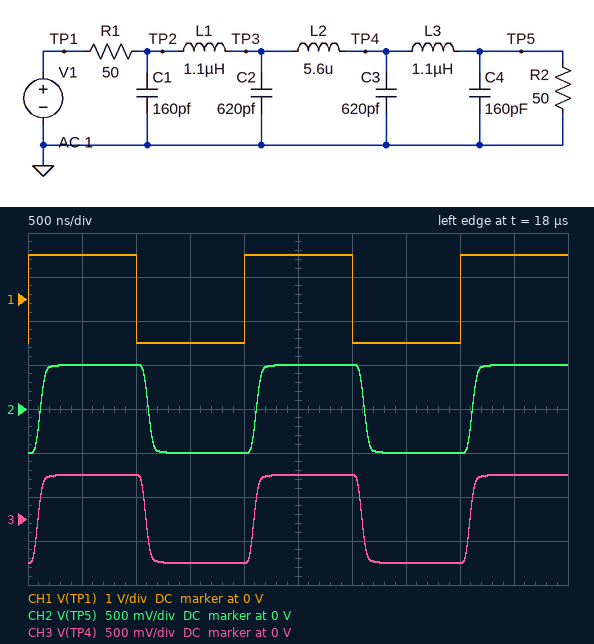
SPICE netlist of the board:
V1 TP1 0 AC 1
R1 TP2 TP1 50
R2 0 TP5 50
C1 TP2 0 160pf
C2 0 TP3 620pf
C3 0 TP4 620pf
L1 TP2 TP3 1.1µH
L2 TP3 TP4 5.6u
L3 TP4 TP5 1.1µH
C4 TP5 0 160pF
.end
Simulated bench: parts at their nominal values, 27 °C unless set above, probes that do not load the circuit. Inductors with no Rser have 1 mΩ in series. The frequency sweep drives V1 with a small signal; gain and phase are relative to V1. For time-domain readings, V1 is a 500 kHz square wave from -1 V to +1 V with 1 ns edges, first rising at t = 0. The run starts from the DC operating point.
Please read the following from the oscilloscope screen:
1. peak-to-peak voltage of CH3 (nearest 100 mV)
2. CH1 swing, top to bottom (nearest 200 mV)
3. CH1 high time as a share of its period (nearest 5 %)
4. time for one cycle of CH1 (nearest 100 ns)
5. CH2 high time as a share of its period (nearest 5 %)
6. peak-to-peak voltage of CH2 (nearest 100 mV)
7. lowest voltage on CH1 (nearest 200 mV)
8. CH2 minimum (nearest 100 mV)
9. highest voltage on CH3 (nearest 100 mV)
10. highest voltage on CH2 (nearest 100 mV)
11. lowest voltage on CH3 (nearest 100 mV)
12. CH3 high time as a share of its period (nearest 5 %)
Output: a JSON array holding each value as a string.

["1.0 V", "2.0 V", "50 %", "2.0 µs", "50 %", "1.0 V", "-1.0 V", "-500 mV", "500 mV", "500 mV", "-500 mV", "50 %"]
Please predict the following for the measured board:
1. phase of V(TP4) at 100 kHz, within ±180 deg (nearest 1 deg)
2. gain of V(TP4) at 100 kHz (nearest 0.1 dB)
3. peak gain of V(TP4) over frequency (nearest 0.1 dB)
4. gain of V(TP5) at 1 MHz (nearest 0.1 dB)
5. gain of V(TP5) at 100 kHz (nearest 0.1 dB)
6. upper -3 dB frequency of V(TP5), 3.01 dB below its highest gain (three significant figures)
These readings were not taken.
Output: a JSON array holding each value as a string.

["-3 deg", "-6.0 dB", "-6.0 dB", "-6.3 dB", "-6.0 dB", "3.71 MHz"]
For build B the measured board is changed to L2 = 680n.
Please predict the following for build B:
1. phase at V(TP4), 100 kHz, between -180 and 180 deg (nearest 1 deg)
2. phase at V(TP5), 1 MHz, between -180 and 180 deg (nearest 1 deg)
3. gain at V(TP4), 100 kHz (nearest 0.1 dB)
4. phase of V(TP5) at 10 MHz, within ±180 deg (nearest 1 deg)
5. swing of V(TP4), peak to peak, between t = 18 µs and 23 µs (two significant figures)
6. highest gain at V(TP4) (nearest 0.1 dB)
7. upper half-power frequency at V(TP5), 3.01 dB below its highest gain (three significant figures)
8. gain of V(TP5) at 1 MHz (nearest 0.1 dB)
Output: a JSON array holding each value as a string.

["-2 deg", "-24 deg", "-6.0 dB", "109 deg", "1.4 V", "-1.3 dB", "13.2 MHz", "-6.0 dB"]
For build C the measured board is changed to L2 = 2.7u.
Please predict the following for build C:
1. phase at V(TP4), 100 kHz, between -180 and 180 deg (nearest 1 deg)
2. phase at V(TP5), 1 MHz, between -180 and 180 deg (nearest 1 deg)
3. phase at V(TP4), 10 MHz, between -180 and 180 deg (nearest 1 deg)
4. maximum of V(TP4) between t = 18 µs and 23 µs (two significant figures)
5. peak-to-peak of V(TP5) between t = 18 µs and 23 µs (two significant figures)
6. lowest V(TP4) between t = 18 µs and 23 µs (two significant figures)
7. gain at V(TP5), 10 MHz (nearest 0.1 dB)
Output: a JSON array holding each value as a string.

["-2 deg", "-32 deg", "67 deg", "640 mV", "1.2 V", "-640 mV", "-18.8 dB"]
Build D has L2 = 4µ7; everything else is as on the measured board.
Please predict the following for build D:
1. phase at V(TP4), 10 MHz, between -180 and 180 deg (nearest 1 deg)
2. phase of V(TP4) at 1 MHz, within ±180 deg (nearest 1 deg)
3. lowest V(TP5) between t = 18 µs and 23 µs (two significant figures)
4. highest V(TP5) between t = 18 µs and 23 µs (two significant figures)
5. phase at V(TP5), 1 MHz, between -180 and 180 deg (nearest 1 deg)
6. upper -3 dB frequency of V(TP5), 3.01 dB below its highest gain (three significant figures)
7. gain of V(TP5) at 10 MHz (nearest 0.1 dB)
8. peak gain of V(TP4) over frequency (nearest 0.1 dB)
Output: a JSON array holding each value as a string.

["60 deg", "-31 deg", "-510 mV", "510 mV", "-39 deg", "4.53 MHz", "-25.5 dB", "-6.0 dB"]
